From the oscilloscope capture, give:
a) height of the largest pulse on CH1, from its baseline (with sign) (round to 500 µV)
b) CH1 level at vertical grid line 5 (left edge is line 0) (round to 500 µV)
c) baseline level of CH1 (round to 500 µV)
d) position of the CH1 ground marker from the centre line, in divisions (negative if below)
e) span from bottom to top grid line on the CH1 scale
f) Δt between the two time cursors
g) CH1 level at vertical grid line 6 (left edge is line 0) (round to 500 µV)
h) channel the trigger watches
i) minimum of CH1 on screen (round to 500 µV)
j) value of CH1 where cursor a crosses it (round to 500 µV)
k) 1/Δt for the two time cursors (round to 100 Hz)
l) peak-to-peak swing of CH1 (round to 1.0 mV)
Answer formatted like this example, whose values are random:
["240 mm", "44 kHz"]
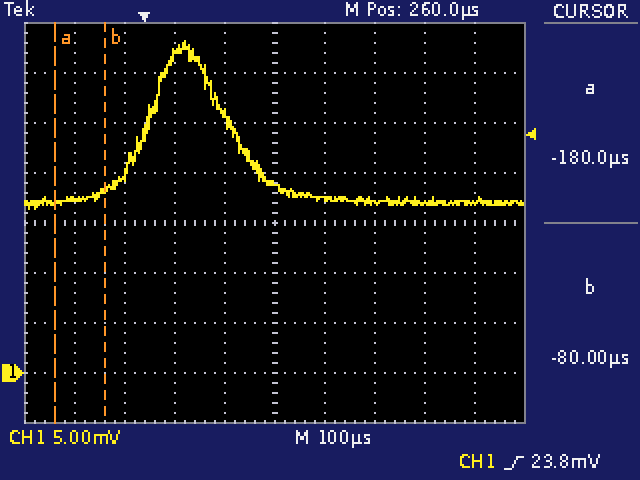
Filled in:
["+16.0 mV", "19.0 mV", "17.0 mV", "-3.0 div", "40 mV", "100 µs", "17.5 mV", "CH1", "16.5 mV", "17.0 mV", "10.0 kHz", "17.0 mV"]
